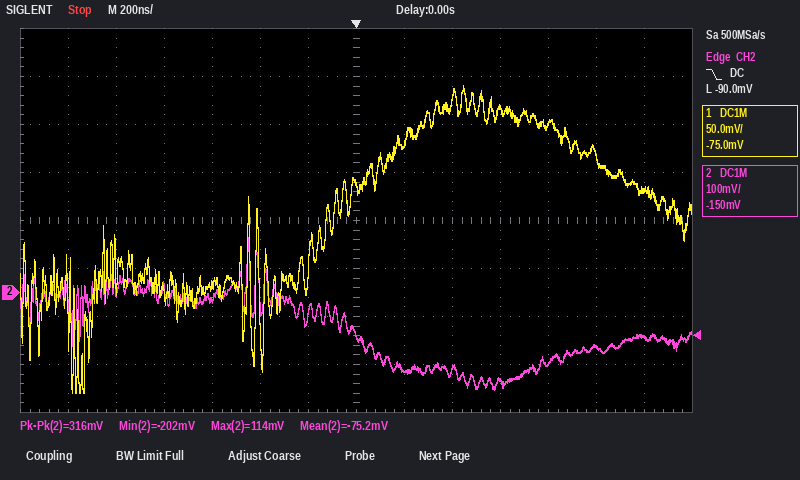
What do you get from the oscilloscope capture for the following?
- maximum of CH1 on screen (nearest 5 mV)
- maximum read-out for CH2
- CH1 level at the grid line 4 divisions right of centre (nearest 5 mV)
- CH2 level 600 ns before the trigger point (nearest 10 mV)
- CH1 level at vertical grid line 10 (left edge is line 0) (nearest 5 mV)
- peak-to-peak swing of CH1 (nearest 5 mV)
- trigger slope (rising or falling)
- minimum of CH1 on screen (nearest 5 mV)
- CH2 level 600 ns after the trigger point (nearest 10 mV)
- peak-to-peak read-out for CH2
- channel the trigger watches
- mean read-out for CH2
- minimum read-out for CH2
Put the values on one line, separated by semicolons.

215 mV; 114 mV; 175 mV; -10 mV; 190 mV; 320 mV; falling; -105 mV; -180 mV; 316 mV; CH2; -75.2 mV; -202 mV
